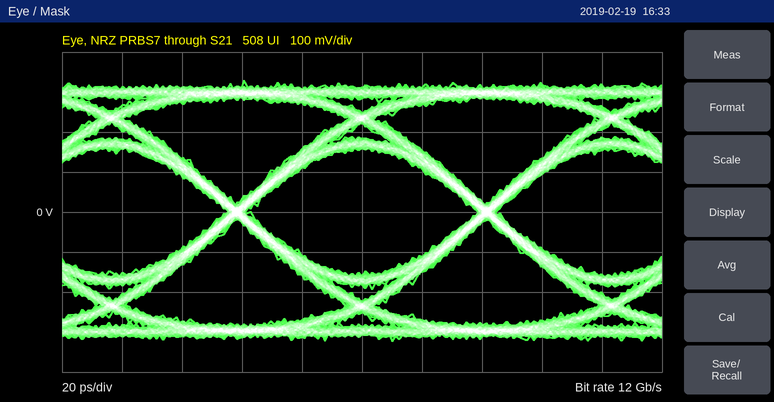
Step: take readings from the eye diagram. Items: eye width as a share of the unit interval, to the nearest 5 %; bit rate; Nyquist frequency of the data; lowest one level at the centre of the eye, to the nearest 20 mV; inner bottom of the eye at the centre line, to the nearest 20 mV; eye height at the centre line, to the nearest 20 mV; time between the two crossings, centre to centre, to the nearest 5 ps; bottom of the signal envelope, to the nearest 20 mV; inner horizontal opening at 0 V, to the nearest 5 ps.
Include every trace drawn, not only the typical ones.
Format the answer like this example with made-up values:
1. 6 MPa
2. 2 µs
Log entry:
1. 90 %
2. 12 Gb/s
3. 6 GHz
4. 160 mV
5. -160 mV
6. 320 mV
7. 85 ps
8. -320 mV
9. 75 ps
